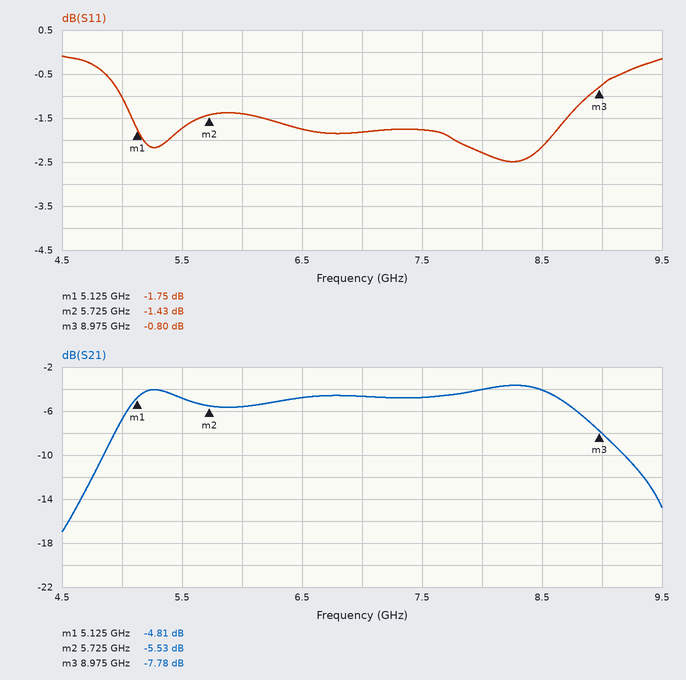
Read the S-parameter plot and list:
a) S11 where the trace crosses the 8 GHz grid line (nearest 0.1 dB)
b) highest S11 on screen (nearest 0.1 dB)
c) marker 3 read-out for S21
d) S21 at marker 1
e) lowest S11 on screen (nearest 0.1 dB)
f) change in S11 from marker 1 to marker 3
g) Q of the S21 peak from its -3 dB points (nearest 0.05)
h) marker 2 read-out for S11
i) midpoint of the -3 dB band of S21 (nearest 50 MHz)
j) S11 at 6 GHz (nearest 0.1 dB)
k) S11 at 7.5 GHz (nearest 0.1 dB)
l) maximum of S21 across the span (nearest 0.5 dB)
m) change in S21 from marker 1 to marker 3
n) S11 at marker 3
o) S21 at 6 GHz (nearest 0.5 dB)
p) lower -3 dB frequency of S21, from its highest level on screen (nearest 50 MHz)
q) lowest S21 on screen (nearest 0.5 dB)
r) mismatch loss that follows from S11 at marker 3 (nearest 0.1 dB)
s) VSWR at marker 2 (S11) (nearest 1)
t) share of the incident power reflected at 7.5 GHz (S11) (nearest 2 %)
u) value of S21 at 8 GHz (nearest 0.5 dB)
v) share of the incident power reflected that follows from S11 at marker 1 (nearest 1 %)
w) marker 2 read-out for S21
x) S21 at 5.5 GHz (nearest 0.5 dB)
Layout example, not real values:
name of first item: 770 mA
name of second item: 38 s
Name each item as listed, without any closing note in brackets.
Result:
S11 where the trace crosses the 8 GHz grid line: -2.3 dB
highest S11 on screen: -0.1 dB
marker 3 read-out for S21: -7.78 dB
S21 at marker 1: -4.81 dB
lowest S11 on screen: -2.5 dB
change in S11 from marker 1 to marker 3: 0.95 dB
Q of the S21 peak from its -3 dB points: 1.80
marker 2 read-out for S11: -1.43 dB
midpoint of the -3 dB band of S21: 6.95 GHz
S11 at 6 GHz: -1.4 dB
S11 at 7.5 GHz: -1.8 dB
maximum of S21 across the span: -3.5 dB
change in S21 from marker 1 to marker 3: -2.97 dB
S11 at marker 3: -0.80 dB
S21 at 6 GHz: -5.5 dB
lower -3 dB frequency of S21, from its highest level on screen: 5.00 GHz
lowest S21 on screen: -17.0 dB
mismatch loss that follows from S11 at marker 3: 7.7 dB
VSWR at marker 2 (S11): 12
share of the incident power reflected at 7.5 GHz (S11): 66 %
value of S21 at 8 GHz: -4.0 dB
share of the incident power reflected that follows from S11 at marker 1: 67 %
marker 2 read-out for S21: -5.53 dB
S21 at 5.5 GHz: -5.0 dB
